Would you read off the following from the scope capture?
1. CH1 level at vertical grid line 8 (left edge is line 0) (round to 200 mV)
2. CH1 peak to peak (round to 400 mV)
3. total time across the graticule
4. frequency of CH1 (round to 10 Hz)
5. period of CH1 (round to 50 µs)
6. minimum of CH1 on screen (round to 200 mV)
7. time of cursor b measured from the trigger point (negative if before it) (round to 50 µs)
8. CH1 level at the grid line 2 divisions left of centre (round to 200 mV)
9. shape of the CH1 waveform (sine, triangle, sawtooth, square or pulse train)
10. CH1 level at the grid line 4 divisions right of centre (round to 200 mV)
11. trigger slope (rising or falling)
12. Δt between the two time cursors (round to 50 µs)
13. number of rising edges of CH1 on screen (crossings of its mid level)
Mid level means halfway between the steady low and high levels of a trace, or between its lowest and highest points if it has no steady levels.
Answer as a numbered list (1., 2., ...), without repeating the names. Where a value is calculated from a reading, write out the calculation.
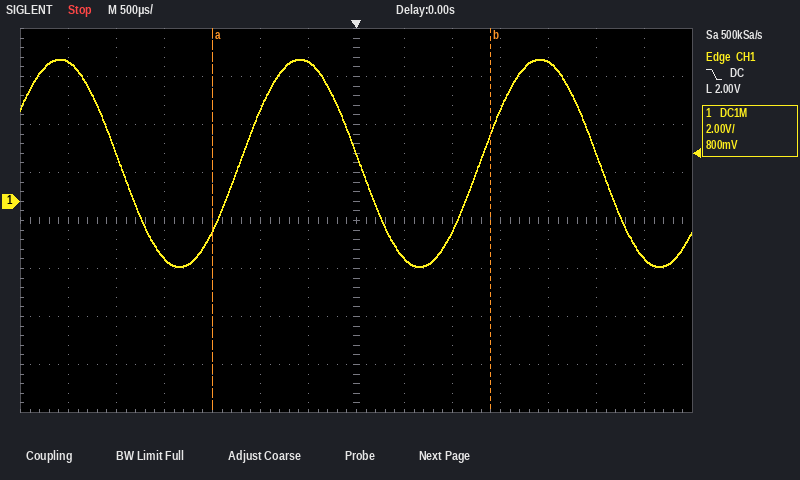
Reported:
1. -2.4 V
2. 8.8 V
3. 7 ms
4. 1 / 2.50 ms ≈ 400 Hz
5. 2.50 ms
6. -2.8 V
7. +1.40 ms
8. 3.8 V
9. sine
10. 5.8 V
11. falling
12. 2.90 ms
13. 2
